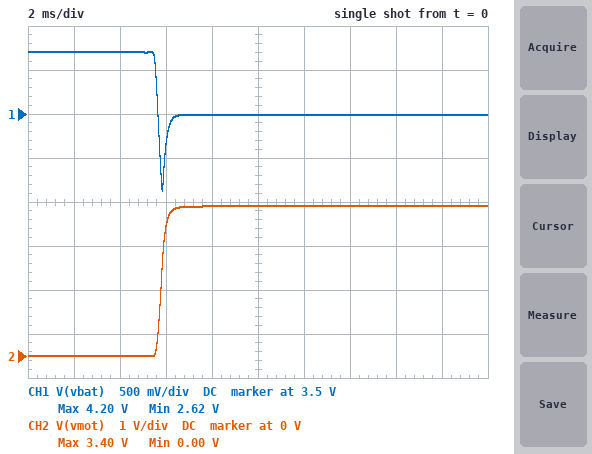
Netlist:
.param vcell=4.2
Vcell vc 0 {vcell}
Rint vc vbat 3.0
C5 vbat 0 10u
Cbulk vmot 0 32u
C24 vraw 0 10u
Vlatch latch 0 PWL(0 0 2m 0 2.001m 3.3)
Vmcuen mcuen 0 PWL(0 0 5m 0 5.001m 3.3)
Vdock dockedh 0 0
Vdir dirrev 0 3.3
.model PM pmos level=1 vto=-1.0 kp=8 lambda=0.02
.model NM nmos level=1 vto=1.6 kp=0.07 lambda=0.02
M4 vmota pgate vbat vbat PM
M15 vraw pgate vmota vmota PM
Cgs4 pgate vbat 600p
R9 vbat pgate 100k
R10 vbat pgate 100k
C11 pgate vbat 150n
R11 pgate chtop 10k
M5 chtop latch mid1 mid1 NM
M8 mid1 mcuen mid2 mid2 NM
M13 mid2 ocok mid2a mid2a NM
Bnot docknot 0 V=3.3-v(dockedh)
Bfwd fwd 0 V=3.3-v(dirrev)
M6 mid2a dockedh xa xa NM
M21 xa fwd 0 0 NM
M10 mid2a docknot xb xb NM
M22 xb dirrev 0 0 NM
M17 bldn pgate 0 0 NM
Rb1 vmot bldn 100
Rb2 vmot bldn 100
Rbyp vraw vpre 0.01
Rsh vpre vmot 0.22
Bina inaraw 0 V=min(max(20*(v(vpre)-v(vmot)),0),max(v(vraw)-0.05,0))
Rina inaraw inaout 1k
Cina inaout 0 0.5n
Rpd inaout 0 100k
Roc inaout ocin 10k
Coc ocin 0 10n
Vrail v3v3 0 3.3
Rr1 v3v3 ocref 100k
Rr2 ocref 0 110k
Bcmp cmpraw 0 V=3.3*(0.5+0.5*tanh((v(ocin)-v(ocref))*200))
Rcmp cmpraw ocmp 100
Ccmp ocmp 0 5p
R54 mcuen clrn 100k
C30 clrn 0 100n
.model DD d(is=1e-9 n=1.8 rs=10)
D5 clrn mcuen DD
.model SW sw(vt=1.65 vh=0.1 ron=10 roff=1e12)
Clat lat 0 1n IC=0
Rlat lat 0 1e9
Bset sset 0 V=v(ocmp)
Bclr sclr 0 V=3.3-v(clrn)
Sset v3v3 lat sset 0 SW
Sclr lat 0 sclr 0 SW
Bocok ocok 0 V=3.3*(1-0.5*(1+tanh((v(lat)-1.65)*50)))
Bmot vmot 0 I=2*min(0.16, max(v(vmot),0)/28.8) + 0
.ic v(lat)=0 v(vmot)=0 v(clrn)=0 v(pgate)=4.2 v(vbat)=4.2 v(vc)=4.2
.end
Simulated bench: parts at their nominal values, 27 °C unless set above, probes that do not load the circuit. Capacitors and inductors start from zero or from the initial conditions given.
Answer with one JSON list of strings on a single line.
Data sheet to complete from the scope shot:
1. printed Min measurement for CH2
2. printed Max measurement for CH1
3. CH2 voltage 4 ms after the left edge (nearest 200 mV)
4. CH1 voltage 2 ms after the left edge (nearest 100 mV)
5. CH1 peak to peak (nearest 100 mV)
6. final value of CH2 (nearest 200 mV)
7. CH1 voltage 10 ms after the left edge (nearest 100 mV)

["0.00 V", "4.20 V", "0 V", "4.2 V", "1.6 V", "3.4 V", "3.5 V"]
